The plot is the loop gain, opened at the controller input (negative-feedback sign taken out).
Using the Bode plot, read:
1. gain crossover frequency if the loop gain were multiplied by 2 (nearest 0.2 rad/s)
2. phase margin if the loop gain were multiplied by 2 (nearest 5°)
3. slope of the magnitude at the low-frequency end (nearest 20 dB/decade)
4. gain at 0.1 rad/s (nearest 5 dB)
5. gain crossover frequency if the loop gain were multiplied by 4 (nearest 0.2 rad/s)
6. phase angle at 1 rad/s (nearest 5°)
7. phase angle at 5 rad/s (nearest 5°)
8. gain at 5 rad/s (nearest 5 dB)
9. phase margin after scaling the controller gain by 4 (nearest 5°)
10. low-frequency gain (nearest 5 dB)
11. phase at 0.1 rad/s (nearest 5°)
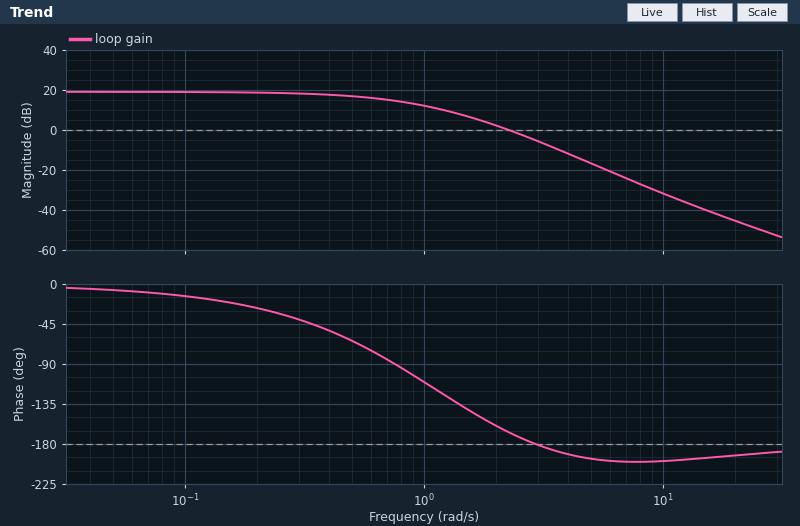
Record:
3.0 rad/s
0°
0 dB/decade
20 dB
4.0 rad/s
-110°
-195°
-15 dB
-10°
20 dB
-15°
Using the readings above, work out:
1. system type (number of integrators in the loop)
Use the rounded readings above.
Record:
0
